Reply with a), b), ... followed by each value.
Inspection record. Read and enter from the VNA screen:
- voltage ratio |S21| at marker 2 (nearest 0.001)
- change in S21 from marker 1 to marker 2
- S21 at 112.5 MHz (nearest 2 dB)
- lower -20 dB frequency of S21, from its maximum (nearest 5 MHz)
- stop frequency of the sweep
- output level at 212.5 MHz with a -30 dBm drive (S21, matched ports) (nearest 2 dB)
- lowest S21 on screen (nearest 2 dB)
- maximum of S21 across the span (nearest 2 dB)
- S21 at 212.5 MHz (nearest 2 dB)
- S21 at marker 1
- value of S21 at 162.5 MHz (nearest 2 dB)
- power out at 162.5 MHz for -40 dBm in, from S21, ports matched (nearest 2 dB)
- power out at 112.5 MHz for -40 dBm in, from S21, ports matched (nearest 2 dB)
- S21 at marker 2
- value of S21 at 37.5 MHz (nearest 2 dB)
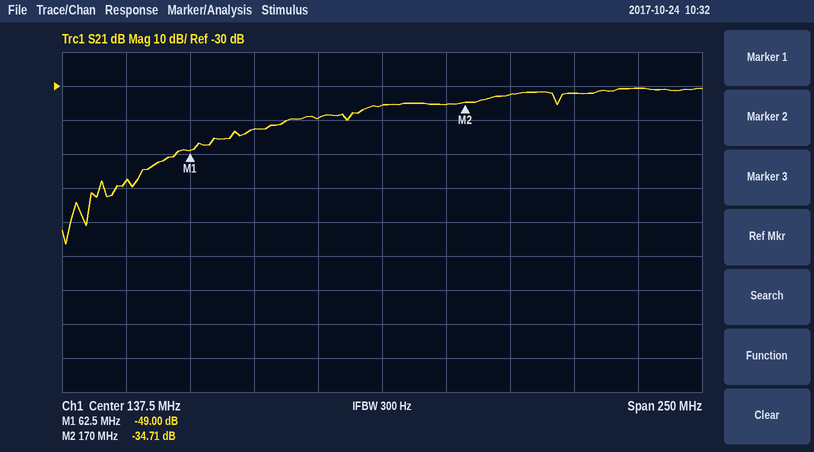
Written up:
a) 0.018
b) 14.29 dB
c) -40 dB
d) 55 MHz
e) 262.5 MHz
f) -62 dBm
g) -76 dB
h) -30 dB
i) -32 dB
j) -49.00 dB
k) -36 dB
l) -76 dBm
m) -80 dBm
n) -34.71 dB
o) -58 dB
